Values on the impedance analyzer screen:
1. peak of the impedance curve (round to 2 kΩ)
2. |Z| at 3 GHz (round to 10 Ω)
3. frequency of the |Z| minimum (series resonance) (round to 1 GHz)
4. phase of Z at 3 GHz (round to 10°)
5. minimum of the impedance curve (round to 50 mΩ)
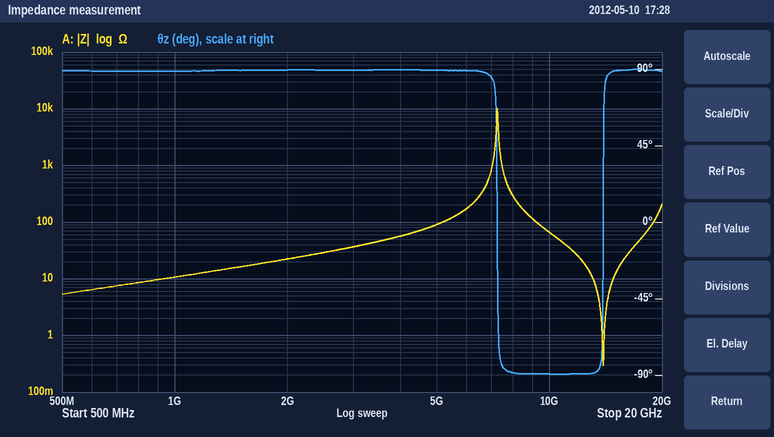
10 kΩ
40 Ω
14 GHz
90°
300 mΩ
